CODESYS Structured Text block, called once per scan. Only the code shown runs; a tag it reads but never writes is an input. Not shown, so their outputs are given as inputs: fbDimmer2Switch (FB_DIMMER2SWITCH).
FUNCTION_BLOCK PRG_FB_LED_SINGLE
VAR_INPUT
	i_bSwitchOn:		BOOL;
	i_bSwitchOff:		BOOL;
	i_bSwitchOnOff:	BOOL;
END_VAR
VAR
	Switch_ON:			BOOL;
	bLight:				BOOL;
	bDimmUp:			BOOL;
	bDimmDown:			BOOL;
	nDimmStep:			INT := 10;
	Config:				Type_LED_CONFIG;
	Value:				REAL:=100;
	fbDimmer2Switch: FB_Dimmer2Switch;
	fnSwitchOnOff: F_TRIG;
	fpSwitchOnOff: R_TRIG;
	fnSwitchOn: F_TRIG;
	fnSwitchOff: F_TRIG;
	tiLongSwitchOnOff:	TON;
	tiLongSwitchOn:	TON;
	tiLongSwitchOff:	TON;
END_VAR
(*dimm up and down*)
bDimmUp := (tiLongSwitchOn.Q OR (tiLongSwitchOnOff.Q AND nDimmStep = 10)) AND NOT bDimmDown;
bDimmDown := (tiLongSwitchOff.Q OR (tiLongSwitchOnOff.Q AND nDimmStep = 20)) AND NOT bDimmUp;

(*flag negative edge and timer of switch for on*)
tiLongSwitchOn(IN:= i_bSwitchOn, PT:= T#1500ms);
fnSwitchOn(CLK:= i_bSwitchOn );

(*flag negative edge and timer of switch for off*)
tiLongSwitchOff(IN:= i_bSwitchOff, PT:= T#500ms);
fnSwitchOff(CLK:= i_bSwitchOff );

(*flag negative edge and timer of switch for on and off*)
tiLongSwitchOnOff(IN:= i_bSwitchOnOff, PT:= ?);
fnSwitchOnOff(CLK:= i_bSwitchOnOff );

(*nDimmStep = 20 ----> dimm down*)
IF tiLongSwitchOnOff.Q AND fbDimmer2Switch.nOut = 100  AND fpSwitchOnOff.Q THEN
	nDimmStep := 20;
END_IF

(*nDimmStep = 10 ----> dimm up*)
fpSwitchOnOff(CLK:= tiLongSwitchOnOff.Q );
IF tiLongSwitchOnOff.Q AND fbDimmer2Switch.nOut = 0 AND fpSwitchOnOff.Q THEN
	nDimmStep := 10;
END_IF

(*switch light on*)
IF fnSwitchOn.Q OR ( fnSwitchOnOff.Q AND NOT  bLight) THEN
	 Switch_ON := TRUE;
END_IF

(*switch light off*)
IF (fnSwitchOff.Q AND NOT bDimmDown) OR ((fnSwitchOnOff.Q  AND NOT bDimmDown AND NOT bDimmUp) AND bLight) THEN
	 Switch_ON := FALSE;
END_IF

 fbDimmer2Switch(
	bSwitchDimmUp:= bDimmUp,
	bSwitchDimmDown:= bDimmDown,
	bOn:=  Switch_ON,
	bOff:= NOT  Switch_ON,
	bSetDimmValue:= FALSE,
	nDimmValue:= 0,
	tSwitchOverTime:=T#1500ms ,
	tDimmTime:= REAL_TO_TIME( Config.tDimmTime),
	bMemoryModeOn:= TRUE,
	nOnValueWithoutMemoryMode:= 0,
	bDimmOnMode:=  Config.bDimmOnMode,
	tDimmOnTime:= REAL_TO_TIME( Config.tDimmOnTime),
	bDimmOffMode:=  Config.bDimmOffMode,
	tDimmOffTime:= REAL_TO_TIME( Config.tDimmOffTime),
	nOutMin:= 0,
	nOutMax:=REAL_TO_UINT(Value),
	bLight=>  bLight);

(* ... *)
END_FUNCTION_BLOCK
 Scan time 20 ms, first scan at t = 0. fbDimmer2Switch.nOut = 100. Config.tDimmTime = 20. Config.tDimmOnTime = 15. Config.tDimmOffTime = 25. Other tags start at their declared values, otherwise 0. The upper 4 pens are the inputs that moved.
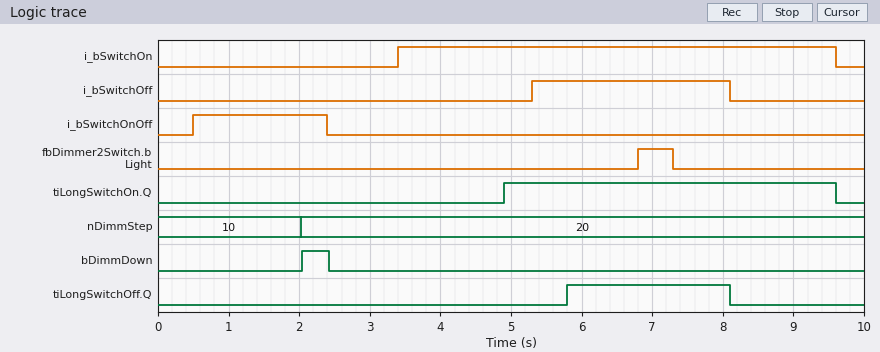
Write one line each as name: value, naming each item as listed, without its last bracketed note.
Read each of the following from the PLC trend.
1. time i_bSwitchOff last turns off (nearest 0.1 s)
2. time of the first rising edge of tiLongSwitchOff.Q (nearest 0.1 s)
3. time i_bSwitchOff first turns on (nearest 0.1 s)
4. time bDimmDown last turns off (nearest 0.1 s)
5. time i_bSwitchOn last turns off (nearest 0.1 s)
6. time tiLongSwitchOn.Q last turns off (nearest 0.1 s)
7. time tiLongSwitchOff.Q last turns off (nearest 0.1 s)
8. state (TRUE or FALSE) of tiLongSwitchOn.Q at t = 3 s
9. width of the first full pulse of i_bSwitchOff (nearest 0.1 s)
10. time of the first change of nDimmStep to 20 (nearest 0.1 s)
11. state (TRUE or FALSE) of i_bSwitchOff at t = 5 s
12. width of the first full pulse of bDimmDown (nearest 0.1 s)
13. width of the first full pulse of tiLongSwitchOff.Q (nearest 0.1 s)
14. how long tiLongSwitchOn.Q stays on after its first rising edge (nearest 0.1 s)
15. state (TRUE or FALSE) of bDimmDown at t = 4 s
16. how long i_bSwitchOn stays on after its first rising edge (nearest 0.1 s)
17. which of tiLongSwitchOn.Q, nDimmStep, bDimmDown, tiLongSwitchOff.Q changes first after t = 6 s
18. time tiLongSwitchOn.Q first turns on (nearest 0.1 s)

time i_bSwitchOff last turns off: 8.1 s
time of the first rising edge of tiLongSwitchOff.Q: 5.8 s
time i_bSwitchOff first turns on: 5.3 s
time bDimmDown last turns off: 2.4 s
time i_bSwitchOn last turns off: 9.6 s
time tiLongSwitchOn.Q last turns off: 9.6 s
time tiLongSwitchOff.Q last turns off: 8.1 s
state (TRUE or FALSE) of tiLongSwitchOn.Q at t = 3 s: FALSE
width of the first full pulse of i_bSwitchOff: 2.8 s
time of the first change of nDimmStep to 20: 2.0 s
state (TRUE or FALSE) of i_bSwitchOff at t = 5 s: FALSE
width of the first full pulse of bDimmDown: 0.4 s
width of the first full pulse of tiLongSwitchOff.Q: 2.3 s
how long tiLongSwitchOn.Q stays on after its first rising edge: 4.7 s
state (TRUE or FALSE) of bDimmDown at t = 4 s: FALSE
how long i_bSwitchOn stays on after its first rising edge: 6.2 s
which of tiLongSwitchOn.Q, nDimmStep, bDimmDown, tiLongSwitchOff.Q changes first after t = 6 s: tiLongSwitchOff.Q
time tiLongSwitchOn.Q first turns on: 4.9 s
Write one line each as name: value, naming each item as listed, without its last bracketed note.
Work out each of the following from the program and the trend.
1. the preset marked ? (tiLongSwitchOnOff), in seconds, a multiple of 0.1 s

the preset marked ? (tiLongSwitchOnOff), in seconds, a multiple of 0.1 s: 1.5 s
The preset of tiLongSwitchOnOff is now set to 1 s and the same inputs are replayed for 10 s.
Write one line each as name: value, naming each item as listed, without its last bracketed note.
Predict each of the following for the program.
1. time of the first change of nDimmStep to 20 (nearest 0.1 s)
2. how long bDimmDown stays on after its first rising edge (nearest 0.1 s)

time of the first change of nDimmStep to 20: 1.5 s
how long bDimmDown stays on after its first rising edge: 0.9 s
